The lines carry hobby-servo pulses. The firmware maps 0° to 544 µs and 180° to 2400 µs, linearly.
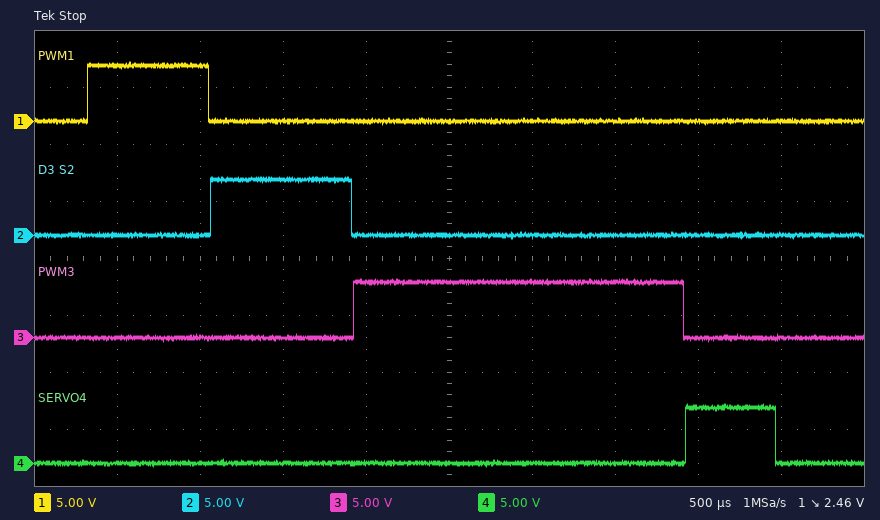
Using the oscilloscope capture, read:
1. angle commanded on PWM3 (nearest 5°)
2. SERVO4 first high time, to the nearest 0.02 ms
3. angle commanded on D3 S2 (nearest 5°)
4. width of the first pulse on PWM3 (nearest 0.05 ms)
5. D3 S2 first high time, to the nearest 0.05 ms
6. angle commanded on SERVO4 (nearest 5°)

140°
0.54 ms
30°
2.00 ms
0.85 ms
0°
